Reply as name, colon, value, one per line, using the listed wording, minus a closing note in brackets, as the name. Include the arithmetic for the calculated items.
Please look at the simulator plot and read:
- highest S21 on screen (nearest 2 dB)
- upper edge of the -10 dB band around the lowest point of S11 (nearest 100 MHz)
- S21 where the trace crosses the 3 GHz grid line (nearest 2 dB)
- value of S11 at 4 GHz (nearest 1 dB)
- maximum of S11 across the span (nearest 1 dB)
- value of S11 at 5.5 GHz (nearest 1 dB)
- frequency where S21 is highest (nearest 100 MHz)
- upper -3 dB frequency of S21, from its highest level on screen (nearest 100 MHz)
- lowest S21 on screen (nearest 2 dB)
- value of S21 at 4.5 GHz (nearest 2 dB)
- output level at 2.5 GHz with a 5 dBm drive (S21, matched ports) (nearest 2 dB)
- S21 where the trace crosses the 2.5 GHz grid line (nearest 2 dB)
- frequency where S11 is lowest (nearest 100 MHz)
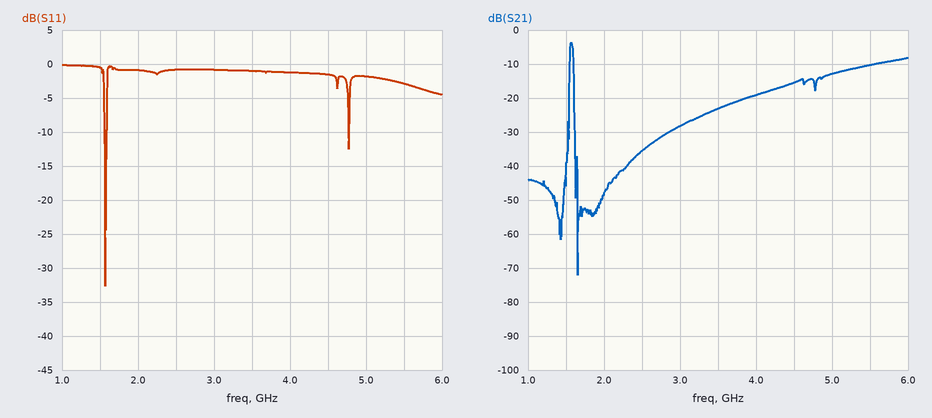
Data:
highest S21 on screen: -4 dB
upper edge of the -10 dB band around the lowest point of S11: 1.6 GHz
S21 where the trace crosses the 3 GHz grid line: -28 dB
value of S11 at 4 GHz: -1 dB
maximum of S11 across the span: 0 dB
value of S11 at 5.5 GHz: -3 dB
frequency where S21 is highest: 1.6 GHz
upper -3 dB frequency of S21, from its highest level on screen: 1.6 GHz
lowest S21 on screen: -72 dB
value of S21 at 4.5 GHz: -16 dB
output level at 2.5 GHz with a 5 dBm drive (S21, matched ports): 5 dBm + (-36 dB) = -30 dBm
S21 where the trace crosses the 2.5 GHz grid line: -36 dB
frequency where S11 is lowest: 1.6 GHz
